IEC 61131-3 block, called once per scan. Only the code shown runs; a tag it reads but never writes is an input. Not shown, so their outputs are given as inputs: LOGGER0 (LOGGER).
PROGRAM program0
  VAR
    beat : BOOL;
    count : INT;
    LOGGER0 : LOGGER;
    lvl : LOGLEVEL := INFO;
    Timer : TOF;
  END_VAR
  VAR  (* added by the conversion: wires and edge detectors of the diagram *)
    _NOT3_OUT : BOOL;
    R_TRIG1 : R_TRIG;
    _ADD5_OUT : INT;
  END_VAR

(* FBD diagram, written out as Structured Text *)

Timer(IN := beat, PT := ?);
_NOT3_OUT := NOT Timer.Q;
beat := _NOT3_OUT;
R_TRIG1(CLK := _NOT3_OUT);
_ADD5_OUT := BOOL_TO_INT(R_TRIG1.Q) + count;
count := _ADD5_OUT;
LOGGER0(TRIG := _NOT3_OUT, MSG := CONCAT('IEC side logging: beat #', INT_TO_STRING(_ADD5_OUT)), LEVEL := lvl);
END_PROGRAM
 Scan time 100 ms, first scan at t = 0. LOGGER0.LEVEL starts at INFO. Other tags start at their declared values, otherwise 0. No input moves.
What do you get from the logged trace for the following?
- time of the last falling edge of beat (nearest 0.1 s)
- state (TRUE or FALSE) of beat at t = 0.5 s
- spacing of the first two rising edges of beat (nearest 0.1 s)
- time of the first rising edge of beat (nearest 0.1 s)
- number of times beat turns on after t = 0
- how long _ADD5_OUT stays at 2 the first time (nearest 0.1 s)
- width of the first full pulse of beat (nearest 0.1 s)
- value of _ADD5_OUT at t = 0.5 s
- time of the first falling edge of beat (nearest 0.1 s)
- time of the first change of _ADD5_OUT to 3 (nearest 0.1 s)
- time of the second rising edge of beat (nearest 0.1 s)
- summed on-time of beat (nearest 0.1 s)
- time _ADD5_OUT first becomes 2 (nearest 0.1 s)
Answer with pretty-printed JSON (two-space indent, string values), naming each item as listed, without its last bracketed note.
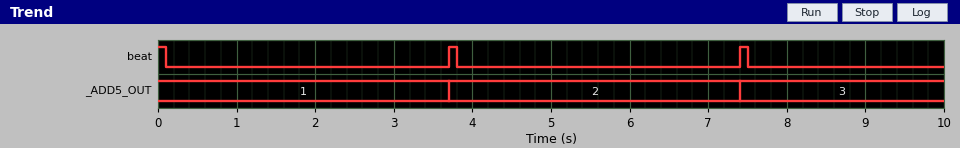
{
  "time of the last falling edge of beat": "7.5 s",
  "state (TRUE or FALSE) of beat at t = 0.5 s": "FALSE",
  "spacing of the first two rising edges of beat": "3.7 s",
  "time of the first rising edge of beat": "3.7 s",
  "number of times beat turns on after t = 0": "2",
  "how long _ADD5_OUT stays at 2 the first time": "3.7 s",
  "width of the first full pulse of beat": "0.1 s",
  "value of _ADD5_OUT at t = 0.5 s": "1",
  "time of the first falling edge of beat": "0.1 s",
  "time of the first change of _ADD5_OUT to 3": "7.4 s",
  "time of the second rising edge of beat": "7.4 s",
  "summed on-time of beat": "0.3 s",
  "time _ADD5_OUT first becomes 2": "3.7 s"
}
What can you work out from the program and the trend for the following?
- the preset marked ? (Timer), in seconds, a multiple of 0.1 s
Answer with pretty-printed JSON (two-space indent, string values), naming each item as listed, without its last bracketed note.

{
  "the preset marked ? (Timer), in seconds, a multiple of 0.1 s": "3.5 s"
}
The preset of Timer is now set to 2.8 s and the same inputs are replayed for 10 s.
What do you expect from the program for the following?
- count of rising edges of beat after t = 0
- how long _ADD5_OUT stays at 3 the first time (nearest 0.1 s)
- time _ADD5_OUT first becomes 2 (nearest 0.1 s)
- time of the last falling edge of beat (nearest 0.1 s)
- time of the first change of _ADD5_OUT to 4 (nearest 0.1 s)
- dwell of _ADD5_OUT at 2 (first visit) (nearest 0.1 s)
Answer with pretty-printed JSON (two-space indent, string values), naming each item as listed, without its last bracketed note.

{
  "count of rising edges of beat after t = 0": "3",
  "how long _ADD5_OUT stays at 3 the first time": "3.0 s",
  "time _ADD5_OUT first becomes 2": "3.0 s",
  "time of the last falling edge of beat": "9.1 s",
  "time of the first change of _ADD5_OUT to 4": "9.0 s",
  "dwell of _ADD5_OUT at 2 (first visit)": "3.0 s"
}
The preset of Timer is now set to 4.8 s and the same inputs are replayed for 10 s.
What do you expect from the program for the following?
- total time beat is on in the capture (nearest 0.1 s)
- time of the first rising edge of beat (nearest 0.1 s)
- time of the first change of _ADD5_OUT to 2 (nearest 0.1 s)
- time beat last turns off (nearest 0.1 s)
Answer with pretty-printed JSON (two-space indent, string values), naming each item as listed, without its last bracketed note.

{
  "total time beat is on in the capture": "0.2 s",
  "time of the first rising edge of beat": "5.0 s",
  "time of the first change of _ADD5_OUT to 2": "5.0 s",
  "time beat last turns off": "5.1 s"
}
